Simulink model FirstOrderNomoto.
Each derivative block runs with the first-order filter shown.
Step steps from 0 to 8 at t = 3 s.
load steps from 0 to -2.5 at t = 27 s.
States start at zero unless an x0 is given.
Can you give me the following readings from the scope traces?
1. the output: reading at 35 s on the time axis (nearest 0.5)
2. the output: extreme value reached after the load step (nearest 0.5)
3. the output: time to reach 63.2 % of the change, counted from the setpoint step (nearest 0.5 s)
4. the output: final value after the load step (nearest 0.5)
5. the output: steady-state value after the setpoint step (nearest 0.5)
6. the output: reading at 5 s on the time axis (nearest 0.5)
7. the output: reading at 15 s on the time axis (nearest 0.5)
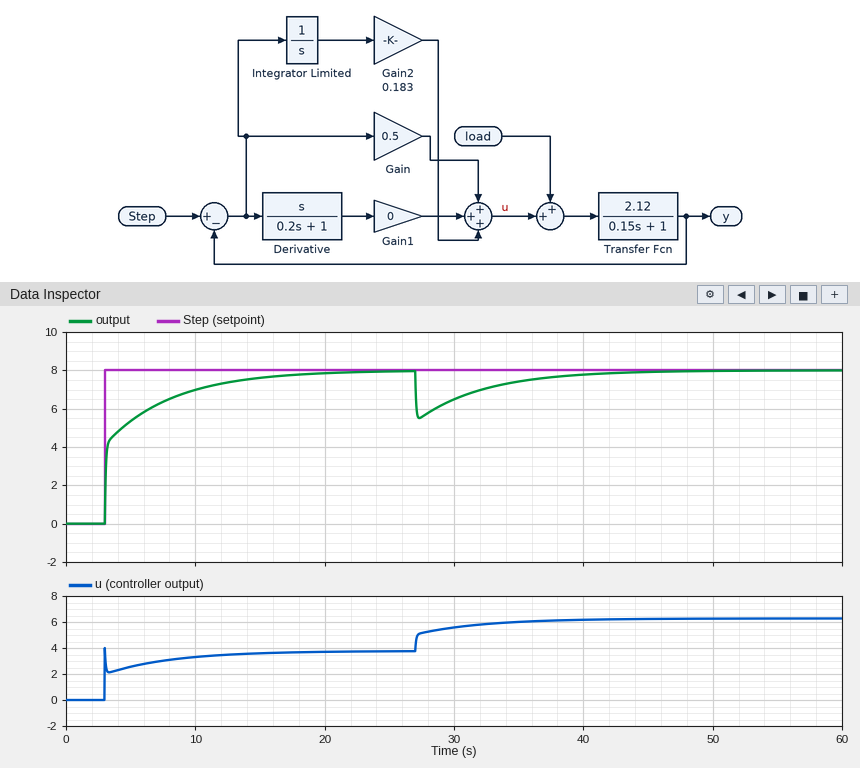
7.5
5.5
1.5 s
8.0
8.0
5.5
7.5
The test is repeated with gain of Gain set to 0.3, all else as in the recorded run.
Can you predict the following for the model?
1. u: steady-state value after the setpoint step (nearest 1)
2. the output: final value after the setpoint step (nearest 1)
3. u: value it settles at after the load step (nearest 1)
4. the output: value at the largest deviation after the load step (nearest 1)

4
8
6
5
